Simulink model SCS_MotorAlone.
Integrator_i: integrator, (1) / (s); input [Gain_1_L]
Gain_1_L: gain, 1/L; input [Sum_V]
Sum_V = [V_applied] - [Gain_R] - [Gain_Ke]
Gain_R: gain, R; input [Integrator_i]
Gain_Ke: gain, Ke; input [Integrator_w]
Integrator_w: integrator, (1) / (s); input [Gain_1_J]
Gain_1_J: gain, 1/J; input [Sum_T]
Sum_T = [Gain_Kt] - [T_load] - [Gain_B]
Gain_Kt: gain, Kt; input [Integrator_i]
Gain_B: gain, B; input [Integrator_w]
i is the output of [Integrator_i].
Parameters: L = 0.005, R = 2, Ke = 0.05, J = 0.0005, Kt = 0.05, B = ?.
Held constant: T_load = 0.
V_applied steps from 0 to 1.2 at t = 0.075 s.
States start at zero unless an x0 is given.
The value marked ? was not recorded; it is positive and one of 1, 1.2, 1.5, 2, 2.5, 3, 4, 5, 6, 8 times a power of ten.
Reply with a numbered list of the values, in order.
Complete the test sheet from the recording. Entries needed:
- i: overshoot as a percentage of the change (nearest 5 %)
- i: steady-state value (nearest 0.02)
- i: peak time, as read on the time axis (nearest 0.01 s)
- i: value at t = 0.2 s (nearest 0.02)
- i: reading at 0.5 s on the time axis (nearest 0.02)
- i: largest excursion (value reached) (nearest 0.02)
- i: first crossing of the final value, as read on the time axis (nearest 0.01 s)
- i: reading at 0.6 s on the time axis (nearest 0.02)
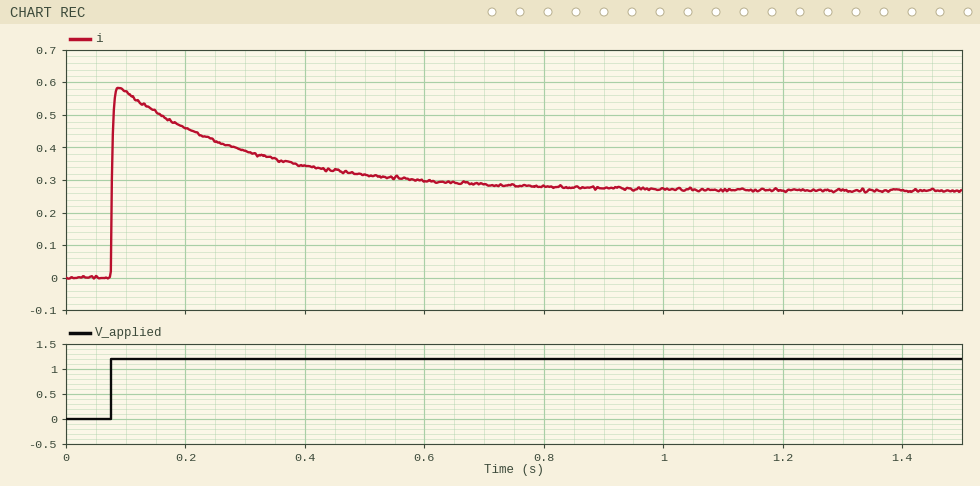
1. 120 %
2. 0.26
3. 0.09 s
4. 0.46
5. 0.32
6. 0.58
7. 0.08 s
8. 0.30
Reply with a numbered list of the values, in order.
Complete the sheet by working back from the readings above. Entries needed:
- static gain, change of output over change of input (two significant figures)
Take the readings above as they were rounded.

1. 0.22
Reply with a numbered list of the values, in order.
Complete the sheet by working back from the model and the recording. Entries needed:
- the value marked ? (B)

1. 0.001
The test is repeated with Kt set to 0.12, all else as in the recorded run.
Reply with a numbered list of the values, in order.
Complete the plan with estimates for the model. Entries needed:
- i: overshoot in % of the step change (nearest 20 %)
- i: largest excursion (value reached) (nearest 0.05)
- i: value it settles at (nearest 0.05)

1. 280 %
2. 0.55
3. 0.15
